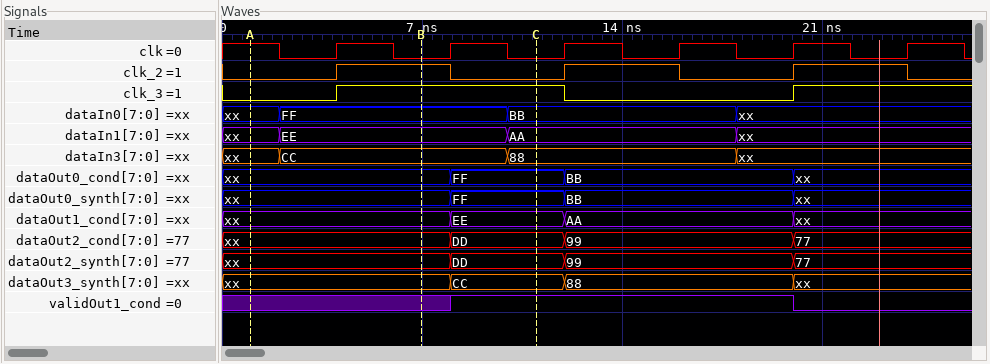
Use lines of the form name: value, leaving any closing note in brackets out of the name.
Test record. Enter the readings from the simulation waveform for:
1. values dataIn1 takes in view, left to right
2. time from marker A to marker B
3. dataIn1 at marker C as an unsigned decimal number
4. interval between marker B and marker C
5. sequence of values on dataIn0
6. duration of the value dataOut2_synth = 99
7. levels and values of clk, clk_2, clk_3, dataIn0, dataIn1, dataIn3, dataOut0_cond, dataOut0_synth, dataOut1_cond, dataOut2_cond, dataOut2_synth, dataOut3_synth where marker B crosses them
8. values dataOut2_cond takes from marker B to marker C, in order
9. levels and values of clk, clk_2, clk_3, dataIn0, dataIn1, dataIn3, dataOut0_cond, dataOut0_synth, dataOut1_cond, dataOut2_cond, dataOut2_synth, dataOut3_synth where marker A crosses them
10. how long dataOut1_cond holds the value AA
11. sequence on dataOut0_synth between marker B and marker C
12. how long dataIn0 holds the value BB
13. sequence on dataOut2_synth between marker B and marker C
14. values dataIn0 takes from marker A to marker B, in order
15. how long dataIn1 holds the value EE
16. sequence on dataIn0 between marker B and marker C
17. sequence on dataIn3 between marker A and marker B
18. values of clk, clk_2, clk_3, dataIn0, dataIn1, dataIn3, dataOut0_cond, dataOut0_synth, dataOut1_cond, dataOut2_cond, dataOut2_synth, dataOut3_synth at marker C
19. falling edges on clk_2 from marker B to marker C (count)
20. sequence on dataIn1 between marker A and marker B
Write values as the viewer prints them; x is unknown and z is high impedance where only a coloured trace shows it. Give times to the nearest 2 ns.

values dataIn1 takes in view, left to right: xx, EE, AA, xx
time from marker A to marker B: 6 ns
dataIn1 at marker C as an unsigned decimal number: 170
interval between marker B and marker C: 4 ns
sequence of values on dataIn0: xx, FF, BB, xx
duration of the value dataOut2_synth = 99: 8 ns
levels and values of clk, clk_2, clk_3, dataIn0, dataIn1, dataIn3, dataOut0_cond, dataOut0_synth, dataOut1_cond, dataOut2_cond, dataOut2_synth, dataOut3_synth where marker B crosses them: clk=0, clk_2=1, clk_3=1, dataIn0=FF, dataIn1=EE, dataIn3=CC, dataOut0_cond=xx, dataOut0_synth=xx, dataOut1_cond=xx, dataOut2_cond=xx, dataOut2_synth=xx, dataOut3_synth=xx
values dataOut2_cond takes from marker B to marker C, in order: xx, DD
levels and values of clk, clk_2, clk_3, dataIn0, dataIn1, dataIn3, dataOut0_cond, dataOut0_synth, dataOut1_cond, dataOut2_cond, dataOut2_synth, dataOut3_synth where marker A crosses them: clk=1, clk_2=0, clk_3=0, dataIn0=xx, dataIn1=xx, dataIn3=xx, dataOut0_cond=xx, dataOut0_synth=xx, dataOut1_cond=xx, dataOut2_cond=xx, dataOut2_synth=xx, dataOut3_synth=xx
how long dataOut1_cond holds the value AA: 8 ns
sequence on dataOut0_synth between marker B and marker C: xx, FF
how long dataIn0 holds the value BB: 8 ns
sequence on dataOut2_synth between marker B and marker C: xx, DD
values dataIn0 takes from marker A to marker B, in order: xx, FF
how long dataIn1 holds the value EE: 8 ns
sequence on dataIn0 between marker B and marker C: FF, BB
sequence on dataIn3 between marker A and marker B: xx, CC
values of clk, clk_2, clk_3, dataIn0, dataIn1, dataIn3, dataOut0_cond, dataOut0_synth, dataOut1_cond, dataOut2_cond, dataOut2_synth, dataOut3_synth at marker C: clk=0, clk_2=0, clk_3=1, dataIn0=BB, dataIn1=AA, dataIn3=88, dataOut0_cond=FF, dataOut0_synth=FF, dataOut1_cond=EE, dataOut2_cond=DD, dataOut2_synth=DD, dataOut3_synth=CC
falling edges on clk_2 from marker B to marker C: 1
sequence on dataIn1 between marker A and marker B: xx, EE
